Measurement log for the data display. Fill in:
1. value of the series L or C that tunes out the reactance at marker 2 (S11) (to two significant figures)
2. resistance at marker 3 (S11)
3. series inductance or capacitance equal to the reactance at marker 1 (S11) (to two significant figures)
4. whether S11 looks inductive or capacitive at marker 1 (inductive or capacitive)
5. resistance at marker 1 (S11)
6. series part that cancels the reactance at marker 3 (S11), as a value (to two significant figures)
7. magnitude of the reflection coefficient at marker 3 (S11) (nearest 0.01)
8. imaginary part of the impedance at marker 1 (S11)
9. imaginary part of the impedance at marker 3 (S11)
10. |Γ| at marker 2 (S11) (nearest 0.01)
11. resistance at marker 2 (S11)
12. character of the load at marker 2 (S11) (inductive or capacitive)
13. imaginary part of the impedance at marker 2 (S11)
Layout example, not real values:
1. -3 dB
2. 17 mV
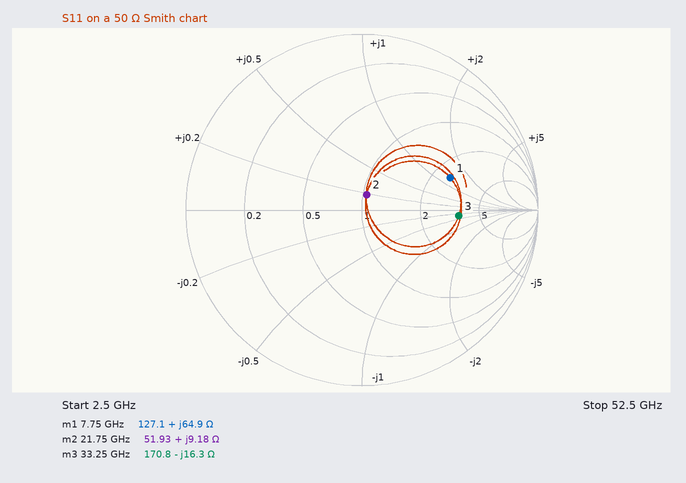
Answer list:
1. 800 fF
2. 170.8 Ω
3. 1.3 nH
4. inductive
5. 127.1 Ω
6. 78 pH
7. 0.55
8. +64.9 Ω
9. -16.3 Ω
10. 0.09
11. 51.93 Ω
12. inductive
13. +9.18 Ω
